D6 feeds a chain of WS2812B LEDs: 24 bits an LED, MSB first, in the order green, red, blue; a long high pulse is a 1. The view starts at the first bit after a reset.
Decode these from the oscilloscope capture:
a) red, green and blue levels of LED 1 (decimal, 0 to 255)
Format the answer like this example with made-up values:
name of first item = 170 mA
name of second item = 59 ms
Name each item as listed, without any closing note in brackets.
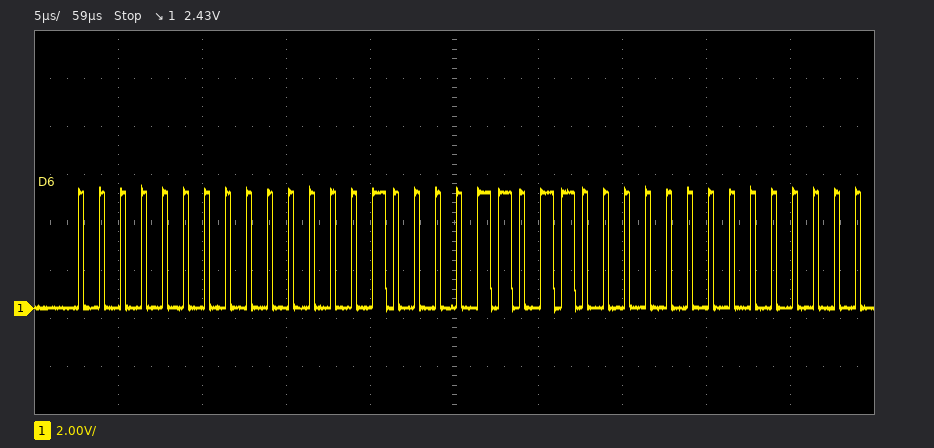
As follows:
red, green and blue levels of LED 1 = 2, 0, 27
